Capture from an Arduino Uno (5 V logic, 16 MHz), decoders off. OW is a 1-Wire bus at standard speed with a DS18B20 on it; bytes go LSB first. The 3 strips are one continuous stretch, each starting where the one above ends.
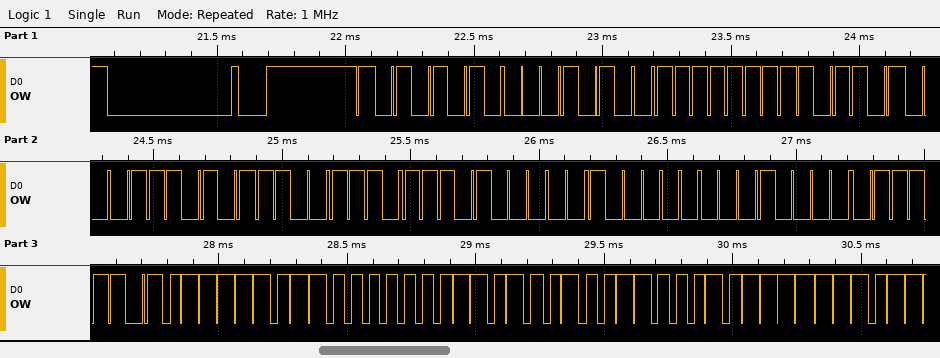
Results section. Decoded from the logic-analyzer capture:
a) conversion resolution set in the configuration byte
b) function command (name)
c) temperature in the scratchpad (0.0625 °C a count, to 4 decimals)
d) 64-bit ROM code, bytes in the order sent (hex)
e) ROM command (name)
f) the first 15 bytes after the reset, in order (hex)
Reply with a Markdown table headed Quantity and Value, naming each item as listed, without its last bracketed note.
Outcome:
| Quantity | Value |
|---|---|
| conversion resolution set in the configuration byte | 12 bits |
| function command | Read Scratchpad |
| temperature in the scratchpad | 27.8750 °C |
| 64-bit ROM code, bytes in the order sent | 28 FF 2D AE 73 17 04 08 |
| ROM command | Match ROM |
| the first 15 bytes after the reset, in order | 55 28 FF 2D AE 73 17 04 08 BE BE 01 4B 46 7F |
